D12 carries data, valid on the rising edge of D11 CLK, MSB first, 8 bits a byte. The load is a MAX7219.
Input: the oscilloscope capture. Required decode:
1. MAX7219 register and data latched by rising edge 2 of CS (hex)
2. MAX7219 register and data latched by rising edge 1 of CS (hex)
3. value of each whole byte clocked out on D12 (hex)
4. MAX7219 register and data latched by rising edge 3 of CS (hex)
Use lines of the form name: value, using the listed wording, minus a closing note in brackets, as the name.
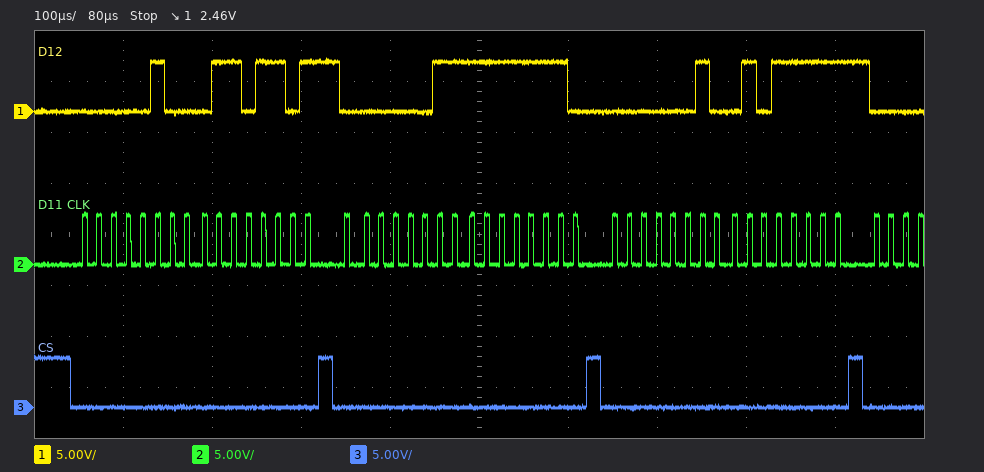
MAX7219 register and data latched by rising edge 2 of CS: register 0x3, data 0xFE
MAX7219 register and data latched by rising edge 1 of CS: register 0x4, data 0x6D
value of each whole byte clocked out on D12: 04 6D 03 FE 02 5F
MAX7219 register and data latched by rising edge 3 of CS: register 0x2, data 0x5F
